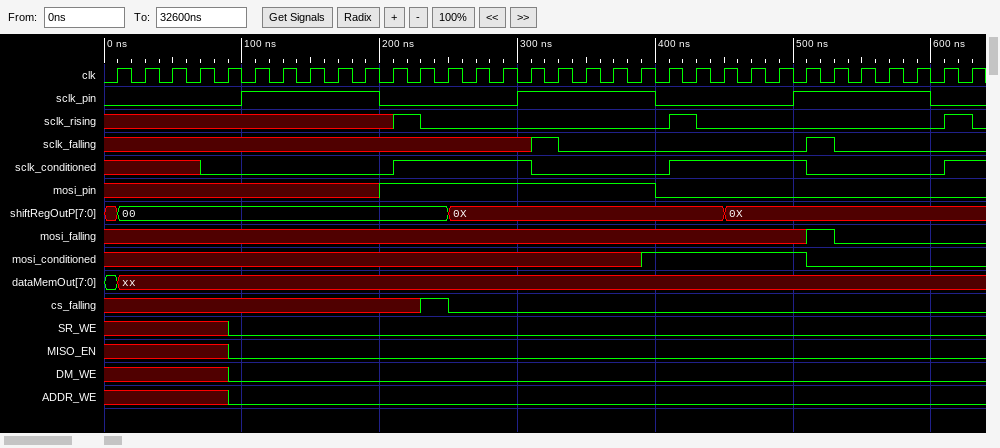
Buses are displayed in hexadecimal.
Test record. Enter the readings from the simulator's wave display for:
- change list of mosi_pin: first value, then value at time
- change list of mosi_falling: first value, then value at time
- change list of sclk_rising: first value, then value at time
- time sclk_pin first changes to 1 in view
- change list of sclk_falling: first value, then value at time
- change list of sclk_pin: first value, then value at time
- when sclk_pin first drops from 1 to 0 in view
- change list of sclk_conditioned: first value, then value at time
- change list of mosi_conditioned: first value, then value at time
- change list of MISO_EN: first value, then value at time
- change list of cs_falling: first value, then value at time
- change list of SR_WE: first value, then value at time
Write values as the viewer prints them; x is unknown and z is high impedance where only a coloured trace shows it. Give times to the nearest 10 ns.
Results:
x, 1 at 200 ns, 0 at 400 ns
x, 1 at 510 ns, 0 at 530 ns
x, 1 at 210 ns, 0 at 230 ns, 1 at 410 ns, 0 at 430 ns, 1 at 610 ns, 0 at 630 ns
100 ns
x, 1 at 310 ns, 0 at 330 ns, 1 at 510 ns, 0 at 530 ns
0, 1 at 100 ns, 0 at 200 ns, 1 at 300 ns, 0 at 400 ns, 1 at 500 ns, 0 at 600 ns
200 ns
x, 0 at 70 ns, 1 at 210 ns, 0 at 310 ns, 1 at 410 ns, 0 at 510 ns, 1 at 610 ns
x, 1 at 390 ns, 0 at 510 ns
x, 0 at 90 ns
x, 1 at 230 ns, 0 at 250 ns
x, 0 at 90 ns
